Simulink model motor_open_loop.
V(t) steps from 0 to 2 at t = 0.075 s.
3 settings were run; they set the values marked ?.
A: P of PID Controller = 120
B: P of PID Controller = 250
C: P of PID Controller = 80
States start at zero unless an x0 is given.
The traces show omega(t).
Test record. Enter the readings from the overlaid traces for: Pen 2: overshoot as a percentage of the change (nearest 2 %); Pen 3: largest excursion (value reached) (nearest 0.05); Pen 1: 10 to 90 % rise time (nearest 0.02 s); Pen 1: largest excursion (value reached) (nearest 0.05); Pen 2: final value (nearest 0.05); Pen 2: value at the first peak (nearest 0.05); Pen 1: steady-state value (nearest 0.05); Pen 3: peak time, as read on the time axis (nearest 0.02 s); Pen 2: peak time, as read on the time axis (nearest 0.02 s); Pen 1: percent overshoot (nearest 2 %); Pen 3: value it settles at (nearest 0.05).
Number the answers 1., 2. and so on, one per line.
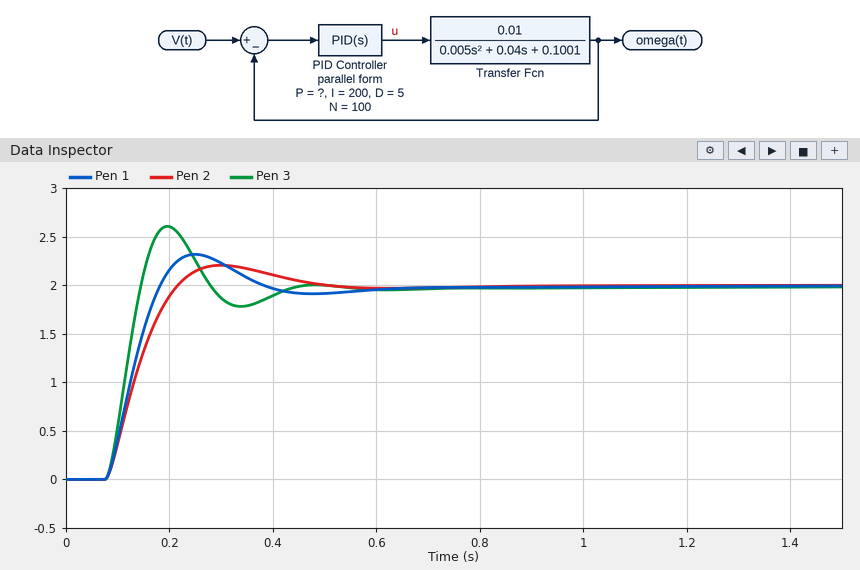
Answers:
1. 10 %
2. 2.60
3. 0.08 s
4. 2.30
5. 2.00
6. 2.20
7. 2.00
8. 0.20 s
9. 0.30 s
10. 16 %
11. 2.00
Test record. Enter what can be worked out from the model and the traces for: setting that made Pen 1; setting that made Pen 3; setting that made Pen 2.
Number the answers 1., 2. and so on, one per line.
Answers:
1. A
2. B
3. C
